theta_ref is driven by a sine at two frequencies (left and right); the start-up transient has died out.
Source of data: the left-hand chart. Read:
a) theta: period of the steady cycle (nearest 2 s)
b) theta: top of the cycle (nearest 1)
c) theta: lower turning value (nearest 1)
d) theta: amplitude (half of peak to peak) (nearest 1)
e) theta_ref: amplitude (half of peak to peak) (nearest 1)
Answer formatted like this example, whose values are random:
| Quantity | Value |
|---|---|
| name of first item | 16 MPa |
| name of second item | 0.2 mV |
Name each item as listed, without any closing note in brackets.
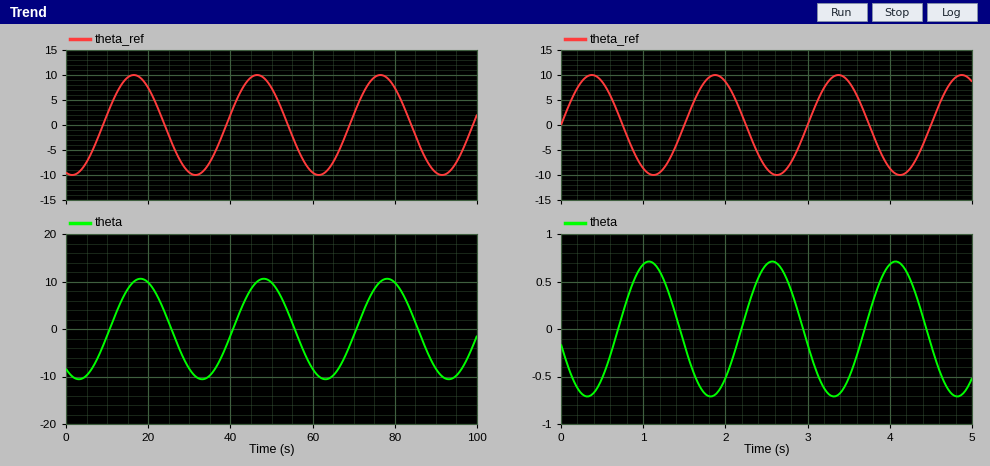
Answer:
| Quantity | Value |
|---|---|
| theta: period of the steady cycle | 30 s |
| theta: top of the cycle | 11 |
| theta: lower turning value | -11 |
| theta: amplitude (half of peak to peak) | 11 |
| theta_ref: amplitude (half of peak to peak) | 10 |
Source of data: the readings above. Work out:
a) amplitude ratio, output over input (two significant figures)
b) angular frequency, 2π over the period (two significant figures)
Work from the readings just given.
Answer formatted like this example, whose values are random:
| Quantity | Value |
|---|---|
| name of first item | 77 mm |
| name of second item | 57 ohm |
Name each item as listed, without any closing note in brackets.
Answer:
| Quantity | Value |
|---|---|
| amplitude ratio, output over input | 1.1 |
| angular frequency, 2π over the period | 0.21 rad/s |
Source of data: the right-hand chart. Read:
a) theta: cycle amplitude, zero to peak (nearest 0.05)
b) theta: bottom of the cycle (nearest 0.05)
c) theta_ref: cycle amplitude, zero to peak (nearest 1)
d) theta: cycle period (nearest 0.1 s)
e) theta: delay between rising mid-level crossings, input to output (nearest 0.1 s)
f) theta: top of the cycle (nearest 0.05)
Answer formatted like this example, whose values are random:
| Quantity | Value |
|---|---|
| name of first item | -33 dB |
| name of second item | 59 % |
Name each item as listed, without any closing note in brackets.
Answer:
| Quantity | Value |
|---|---|
| theta: cycle amplitude, zero to peak | 0.70 |
| theta: bottom of the cycle | -0.70 |
| theta_ref: cycle amplitude, zero to peak | 10 |
| theta: cycle period | 1.5 s |
| theta: delay between rising mid-level crossings, input to output | 0.7 s |
| theta: top of the cycle | 0.70 |
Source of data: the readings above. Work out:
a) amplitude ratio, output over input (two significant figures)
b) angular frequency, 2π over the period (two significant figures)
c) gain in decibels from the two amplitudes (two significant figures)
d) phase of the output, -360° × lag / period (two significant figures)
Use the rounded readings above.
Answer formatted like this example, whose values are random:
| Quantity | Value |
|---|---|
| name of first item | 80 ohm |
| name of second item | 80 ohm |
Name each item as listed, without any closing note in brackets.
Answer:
| Quantity | Value |
|---|---|
| amplitude ratio, output over input | 0.070 |
| angular frequency, 2π over the period | 4.2 rad/s |
| gain in decibels from the two amplitudes | -23 dB |
| phase of the output, -360° × lag / period | -170° |
